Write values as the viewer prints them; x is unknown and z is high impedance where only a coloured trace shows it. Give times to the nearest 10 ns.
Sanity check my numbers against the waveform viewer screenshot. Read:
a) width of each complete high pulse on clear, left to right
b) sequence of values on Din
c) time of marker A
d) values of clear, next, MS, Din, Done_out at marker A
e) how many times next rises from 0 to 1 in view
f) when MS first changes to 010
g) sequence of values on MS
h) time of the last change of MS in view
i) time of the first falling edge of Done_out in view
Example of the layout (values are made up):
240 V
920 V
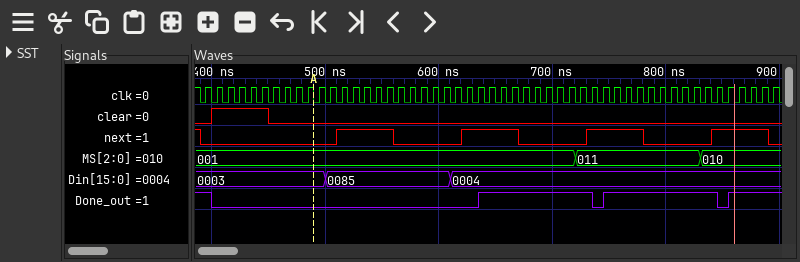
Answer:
50 ns
0003, 0085, 0004
490 ns
clear=0, next=0, MS=001, Din=0003, Done_out=0
4
830 ns
001, 011, 010
830 ns
400 ns
